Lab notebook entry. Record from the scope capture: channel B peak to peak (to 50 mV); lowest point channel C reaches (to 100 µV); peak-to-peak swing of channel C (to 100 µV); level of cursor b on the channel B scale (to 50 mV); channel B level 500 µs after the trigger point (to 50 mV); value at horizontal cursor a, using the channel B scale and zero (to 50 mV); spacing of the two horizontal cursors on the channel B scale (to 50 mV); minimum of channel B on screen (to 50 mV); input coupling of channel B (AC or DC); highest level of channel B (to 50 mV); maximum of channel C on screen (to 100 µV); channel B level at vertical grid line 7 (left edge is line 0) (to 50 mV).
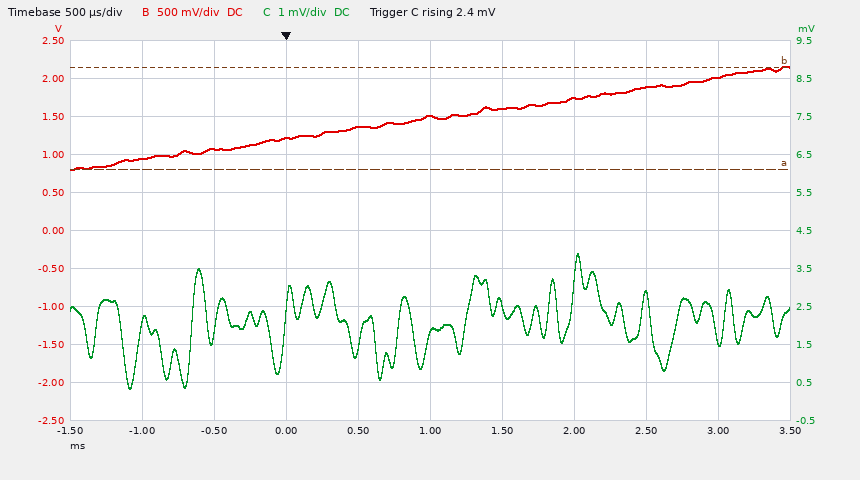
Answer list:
1.35 V
300 µV
3.6 mV
2.15 V
1.35 V
800 mV
1.35 V
800 mV
DC
2.15 V
3.9 mV
1.75 V
